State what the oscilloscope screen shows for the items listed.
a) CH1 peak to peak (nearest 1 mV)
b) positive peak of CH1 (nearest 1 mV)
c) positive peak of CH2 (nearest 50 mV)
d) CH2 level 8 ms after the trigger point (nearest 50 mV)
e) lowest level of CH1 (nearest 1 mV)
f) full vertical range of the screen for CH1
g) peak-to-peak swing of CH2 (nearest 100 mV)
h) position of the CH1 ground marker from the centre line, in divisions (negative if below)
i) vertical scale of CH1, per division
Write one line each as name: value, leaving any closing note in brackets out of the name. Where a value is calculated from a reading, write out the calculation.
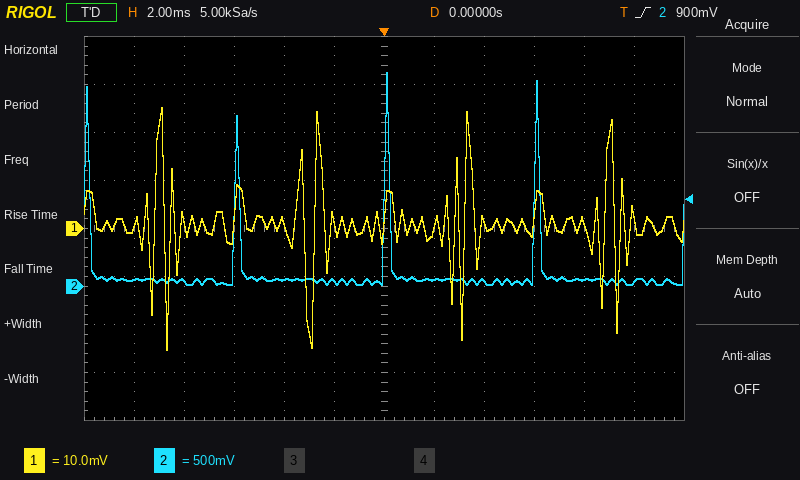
CH1 peak to peak: 25 mV − (-25 mV) = 50 mV
positive peak of CH1: 25 mV
positive peak of CH2: 2.20 V
CH2 level 8 ms after the trigger point: 50 mV
lowest level of CH1: -25 mV
full vertical range of the screen for CH1: 80 mV
peak-to-peak swing of CH2: 2.20 V
position of the CH1 ground marker from the centre line, in divisions: 0.0 div
vertical scale of CH1, per division: 10 mV
